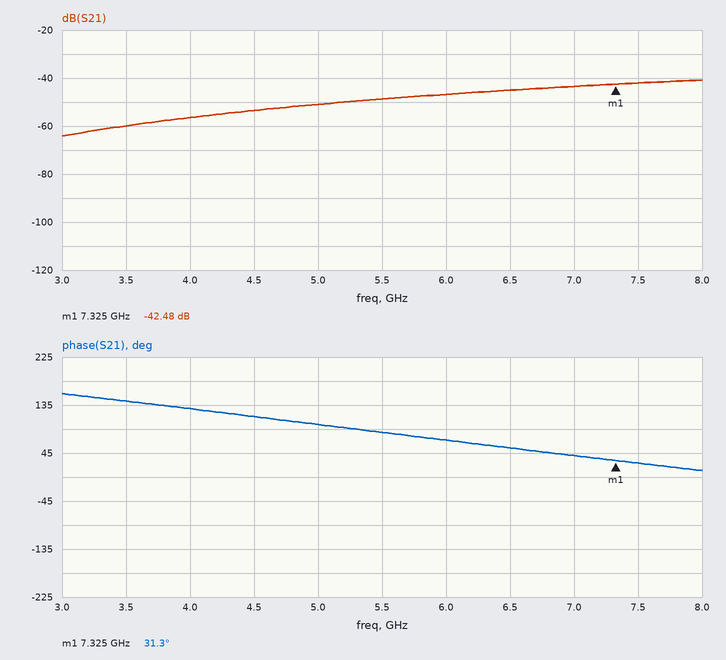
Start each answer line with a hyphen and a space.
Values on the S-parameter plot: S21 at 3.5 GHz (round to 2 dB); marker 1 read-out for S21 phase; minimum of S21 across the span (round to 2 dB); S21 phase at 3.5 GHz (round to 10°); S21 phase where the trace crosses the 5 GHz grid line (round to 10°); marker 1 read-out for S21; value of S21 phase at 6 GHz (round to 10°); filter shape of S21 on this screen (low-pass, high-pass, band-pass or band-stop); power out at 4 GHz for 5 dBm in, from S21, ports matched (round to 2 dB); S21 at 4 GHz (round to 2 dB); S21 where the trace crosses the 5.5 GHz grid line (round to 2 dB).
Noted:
- -60 dB
- 31.3°
- -64 dB
- 140°
- 100°
- -42.48 dB
- 70°
- high-pass
- -52 dBm
- -56 dB
- -48 dB
